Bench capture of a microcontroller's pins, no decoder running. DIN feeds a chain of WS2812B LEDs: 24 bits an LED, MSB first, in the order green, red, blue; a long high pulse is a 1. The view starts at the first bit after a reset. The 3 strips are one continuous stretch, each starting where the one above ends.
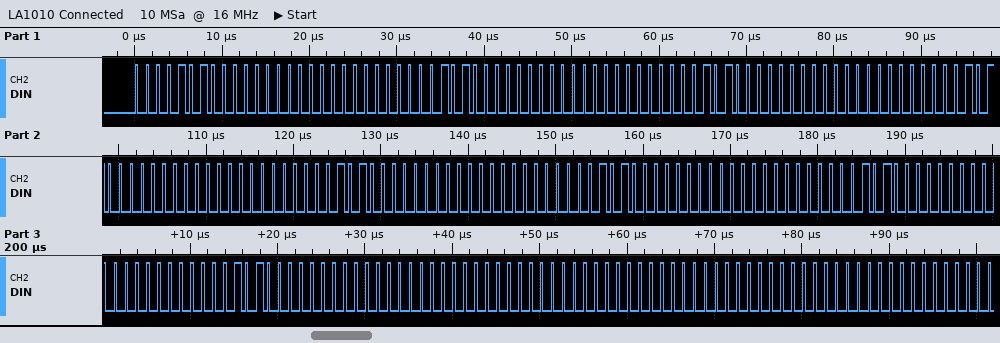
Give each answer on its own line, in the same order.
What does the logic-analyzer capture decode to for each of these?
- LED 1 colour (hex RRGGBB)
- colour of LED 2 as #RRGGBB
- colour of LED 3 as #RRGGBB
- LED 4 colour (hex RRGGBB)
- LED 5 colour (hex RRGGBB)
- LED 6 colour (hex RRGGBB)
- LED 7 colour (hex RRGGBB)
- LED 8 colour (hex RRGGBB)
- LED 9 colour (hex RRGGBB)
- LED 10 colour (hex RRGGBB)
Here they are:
#000A00
#000A00
#000A00
#000A00
#000A00
#000A00
#000A00
#000A00
#000000
#000000
